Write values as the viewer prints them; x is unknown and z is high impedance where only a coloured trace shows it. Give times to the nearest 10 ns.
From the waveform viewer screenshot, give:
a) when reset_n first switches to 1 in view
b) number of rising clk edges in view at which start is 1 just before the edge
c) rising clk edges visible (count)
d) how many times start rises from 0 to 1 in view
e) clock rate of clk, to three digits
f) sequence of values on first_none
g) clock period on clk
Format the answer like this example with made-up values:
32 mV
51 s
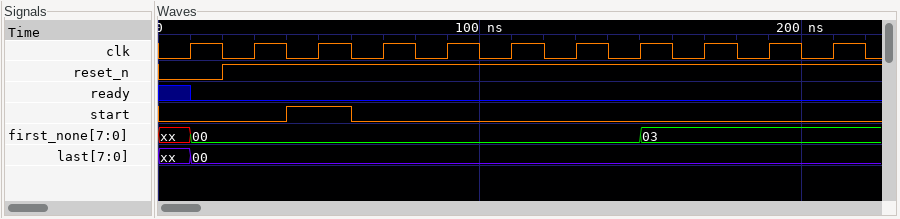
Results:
20 ns
1
11
1
50.0 MHz
xx, 00, 03
20 ns
